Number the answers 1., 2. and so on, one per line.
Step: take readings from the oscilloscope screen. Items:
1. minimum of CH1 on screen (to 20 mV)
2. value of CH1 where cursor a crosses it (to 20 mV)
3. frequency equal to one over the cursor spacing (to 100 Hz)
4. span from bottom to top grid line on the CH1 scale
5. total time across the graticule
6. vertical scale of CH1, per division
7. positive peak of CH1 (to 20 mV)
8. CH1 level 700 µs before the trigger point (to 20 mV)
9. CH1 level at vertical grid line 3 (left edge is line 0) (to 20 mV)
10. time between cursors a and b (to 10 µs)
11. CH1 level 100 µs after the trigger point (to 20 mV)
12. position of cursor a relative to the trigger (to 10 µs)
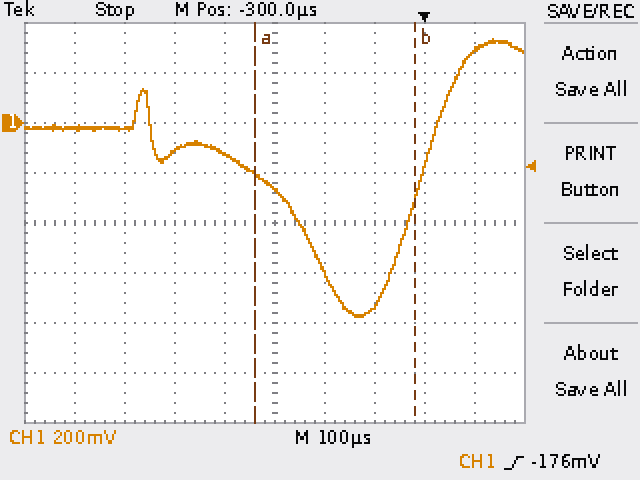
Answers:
1. -780 mV
2. -200 mV
3. 3.1 kHz
4. 1.6 V
5. 1 ms
6. 200 mV
7. 340 mV
8. -20 mV
9. -120 mV
10. 320 µs
11. 280 mV
12. -340 µs
